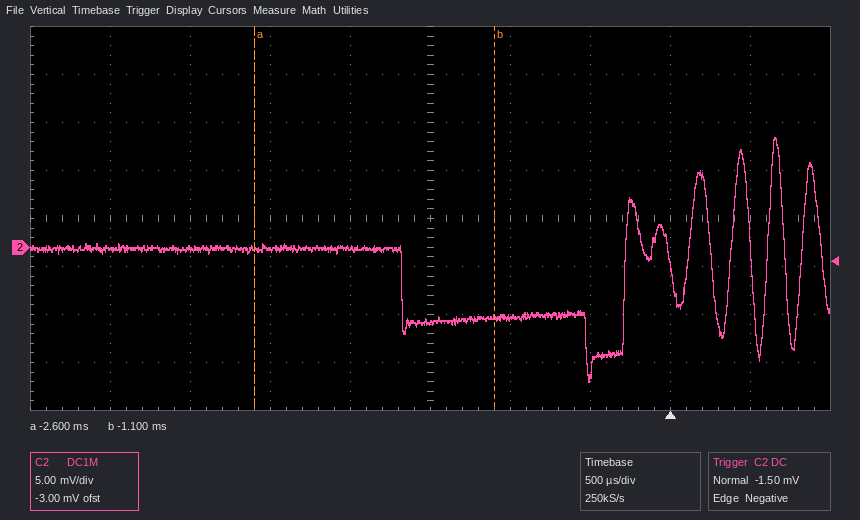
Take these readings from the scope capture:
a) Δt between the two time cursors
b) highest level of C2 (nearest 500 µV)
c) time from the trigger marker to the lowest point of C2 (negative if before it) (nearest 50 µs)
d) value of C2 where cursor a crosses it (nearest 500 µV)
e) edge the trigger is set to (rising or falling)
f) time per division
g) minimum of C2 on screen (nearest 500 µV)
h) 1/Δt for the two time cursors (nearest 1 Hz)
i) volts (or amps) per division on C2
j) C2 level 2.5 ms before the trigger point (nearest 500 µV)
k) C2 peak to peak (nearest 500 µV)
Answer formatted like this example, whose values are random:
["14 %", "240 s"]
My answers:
["1.50 ms", "11.5 mV", "-500 µs", "0.0 mV", "falling", "500 µs", "-14.0 mV", "667 Hz", "5 mV", "0.0 mV", "25.5 mV"]
